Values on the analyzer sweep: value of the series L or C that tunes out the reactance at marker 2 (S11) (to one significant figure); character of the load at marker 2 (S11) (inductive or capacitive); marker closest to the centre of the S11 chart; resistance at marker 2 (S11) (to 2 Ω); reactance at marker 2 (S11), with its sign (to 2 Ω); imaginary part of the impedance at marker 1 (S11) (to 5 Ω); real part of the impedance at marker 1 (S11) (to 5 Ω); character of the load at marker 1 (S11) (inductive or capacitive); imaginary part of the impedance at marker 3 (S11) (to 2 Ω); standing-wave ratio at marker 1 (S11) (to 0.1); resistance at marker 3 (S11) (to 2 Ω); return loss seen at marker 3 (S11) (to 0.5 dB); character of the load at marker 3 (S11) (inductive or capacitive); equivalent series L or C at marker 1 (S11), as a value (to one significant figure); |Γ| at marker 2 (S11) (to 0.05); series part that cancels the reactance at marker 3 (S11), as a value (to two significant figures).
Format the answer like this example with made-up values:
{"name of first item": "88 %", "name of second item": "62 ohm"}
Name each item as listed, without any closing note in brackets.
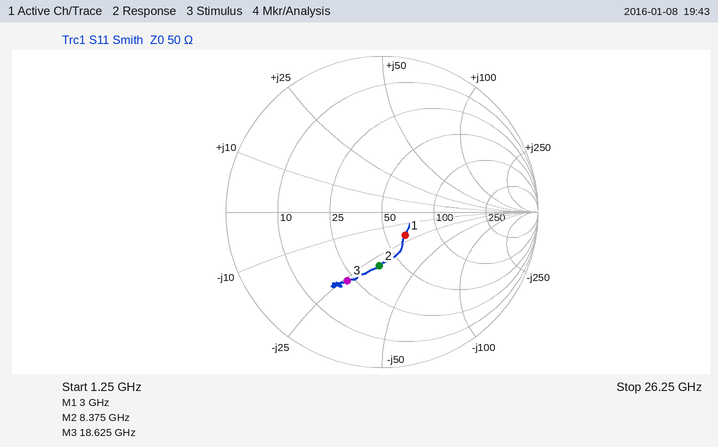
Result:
{"value of the series L or C that tunes out the reactance at marker 2 (S11)": "600 pH", "character of the load at marker 2 (S11)": "capacitive", "marker closest to the centre of the S11 chart": "marker 1", "resistance at marker 2 (S11)": "38 Ω", "reactance at marker 2 (S11), with its sign": "-30 Ω", "imaginary part of the impedance at marker 1 (S11)": "-20 Ω", "real part of the impedance at marker 1 (S11)": "65 Ω", "character of the load at marker 1 (S11)": "capacitive", "imaginary part of the impedance at marker 3 (S11)": "-26 Ω", "standing-wave ratio at marker 1 (S11)": "1.5", "resistance at marker 3 (S11)": "22 Ω", "return loss seen at marker 3 (S11)": "6.0 dB", "character of the load at marker 3 (S11)": "capacitive", "equivalent series L or C at marker 1 (S11), as a value": "3 pF", "|Γ| at marker 2 (S11)": "0.35", "series part that cancels the reactance at marker 3 (S11), as a value": "220 pH"}
